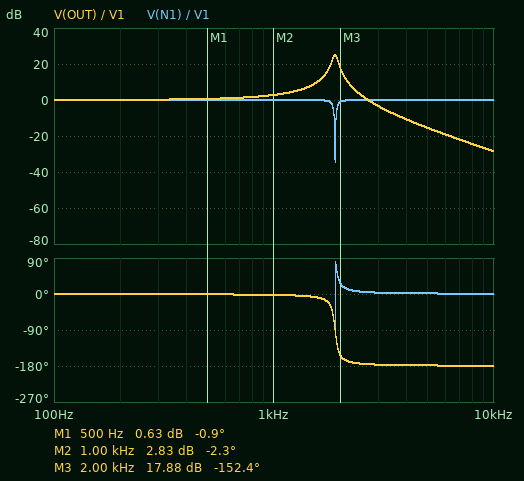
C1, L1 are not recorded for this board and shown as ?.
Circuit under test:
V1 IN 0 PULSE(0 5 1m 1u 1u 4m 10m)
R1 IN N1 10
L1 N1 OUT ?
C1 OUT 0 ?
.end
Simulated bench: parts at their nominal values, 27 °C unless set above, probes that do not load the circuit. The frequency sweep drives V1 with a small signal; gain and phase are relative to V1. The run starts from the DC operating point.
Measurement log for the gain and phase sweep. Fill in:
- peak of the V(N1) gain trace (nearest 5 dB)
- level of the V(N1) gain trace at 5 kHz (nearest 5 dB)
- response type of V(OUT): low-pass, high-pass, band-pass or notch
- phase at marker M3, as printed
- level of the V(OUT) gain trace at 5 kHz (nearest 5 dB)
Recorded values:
0 dB
0 dB
band-pass
-152.4 deg
-15 dB
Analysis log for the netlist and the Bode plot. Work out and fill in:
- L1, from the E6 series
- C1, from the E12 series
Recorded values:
15 mH
470 nF
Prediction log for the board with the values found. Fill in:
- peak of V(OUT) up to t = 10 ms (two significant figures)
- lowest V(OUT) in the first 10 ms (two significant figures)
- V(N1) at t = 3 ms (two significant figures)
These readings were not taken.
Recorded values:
9.6 V
-5.7 V
5.1 V
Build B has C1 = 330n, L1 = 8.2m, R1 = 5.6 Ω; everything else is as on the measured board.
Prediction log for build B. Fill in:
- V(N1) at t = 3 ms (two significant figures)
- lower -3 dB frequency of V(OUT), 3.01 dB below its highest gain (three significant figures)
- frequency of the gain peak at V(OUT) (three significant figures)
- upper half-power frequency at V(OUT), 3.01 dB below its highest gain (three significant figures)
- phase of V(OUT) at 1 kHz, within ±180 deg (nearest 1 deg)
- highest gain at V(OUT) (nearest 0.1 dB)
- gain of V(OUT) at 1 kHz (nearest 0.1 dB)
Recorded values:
4.9 V
3.00 kHz
3.06 kHz
3.11 kHz
-1 deg
29.0 dB
1.0 dB
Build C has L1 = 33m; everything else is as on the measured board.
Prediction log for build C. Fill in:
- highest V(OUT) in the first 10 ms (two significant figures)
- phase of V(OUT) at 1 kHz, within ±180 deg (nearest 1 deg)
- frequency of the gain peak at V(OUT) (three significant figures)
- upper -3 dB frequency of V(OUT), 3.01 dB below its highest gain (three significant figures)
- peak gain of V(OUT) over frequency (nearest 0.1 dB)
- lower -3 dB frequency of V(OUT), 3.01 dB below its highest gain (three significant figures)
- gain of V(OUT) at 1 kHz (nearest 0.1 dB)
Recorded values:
9.7 V
-4 deg
1.28 kHz
1.30 kHz
28.5 dB
1.25 kHz
8.2 dB
